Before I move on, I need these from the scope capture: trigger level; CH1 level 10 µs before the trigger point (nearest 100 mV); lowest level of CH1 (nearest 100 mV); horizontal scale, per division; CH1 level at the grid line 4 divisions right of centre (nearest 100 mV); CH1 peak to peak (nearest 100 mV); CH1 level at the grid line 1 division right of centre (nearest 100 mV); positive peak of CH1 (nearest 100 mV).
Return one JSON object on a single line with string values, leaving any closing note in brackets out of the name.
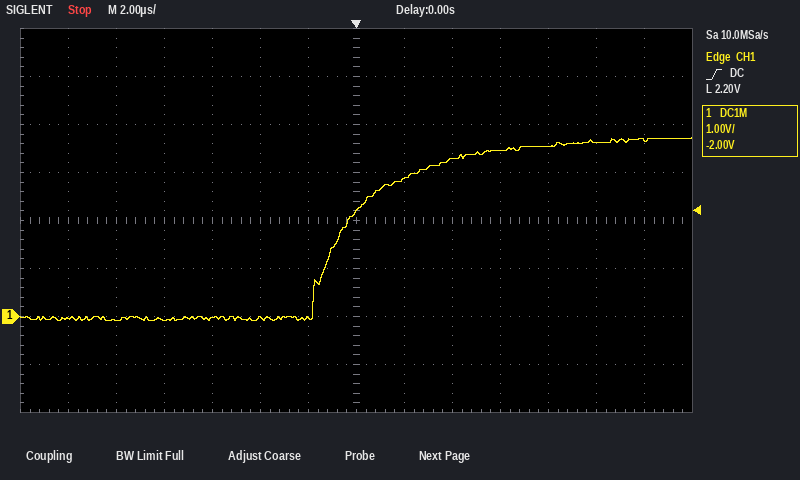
{"trigger level": "2.20 V", "CH1 level 10 µs before the trigger point": "-100 mV", "lowest level of CH1": "-100 mV", "horizontal scale, per division": "2 µs", "CH1 level at the grid line 4 divisions right of centre": "3.5 V", "CH1 peak to peak": "3.8 V", "CH1 level at the grid line 1 division right of centre": "2.9 V", "positive peak of CH1": "3.7 V"}
